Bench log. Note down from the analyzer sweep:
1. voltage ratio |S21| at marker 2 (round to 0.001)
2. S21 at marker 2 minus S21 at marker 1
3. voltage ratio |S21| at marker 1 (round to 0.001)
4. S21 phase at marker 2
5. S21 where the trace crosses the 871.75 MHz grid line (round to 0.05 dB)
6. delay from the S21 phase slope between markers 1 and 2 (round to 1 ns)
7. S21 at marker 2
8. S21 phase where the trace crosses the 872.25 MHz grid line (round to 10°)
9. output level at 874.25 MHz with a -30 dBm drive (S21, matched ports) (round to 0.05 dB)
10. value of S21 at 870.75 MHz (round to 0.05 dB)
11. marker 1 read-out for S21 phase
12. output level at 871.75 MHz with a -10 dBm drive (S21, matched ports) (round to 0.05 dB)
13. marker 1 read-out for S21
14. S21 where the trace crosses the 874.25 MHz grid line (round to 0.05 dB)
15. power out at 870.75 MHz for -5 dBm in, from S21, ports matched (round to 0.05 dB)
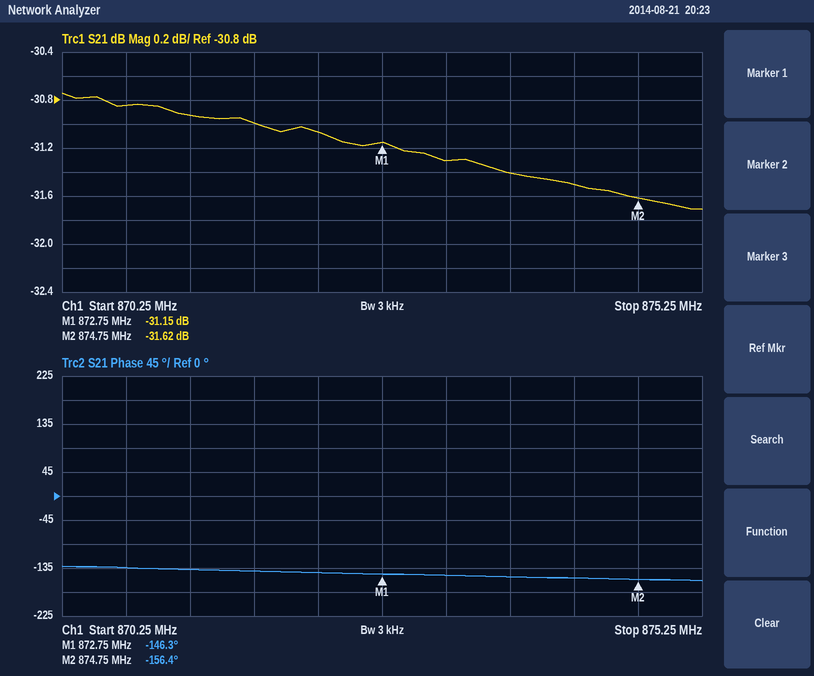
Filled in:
0.026
-0.47 dB
0.028
-156.4°
-31.00 dB
14 ns
-31.62 dB
-140°
-61.50 dBm
-30.85 dB
-146.3°
-41.00 dBm
-31.15 dB
-31.50 dB
-35.85 dBm
